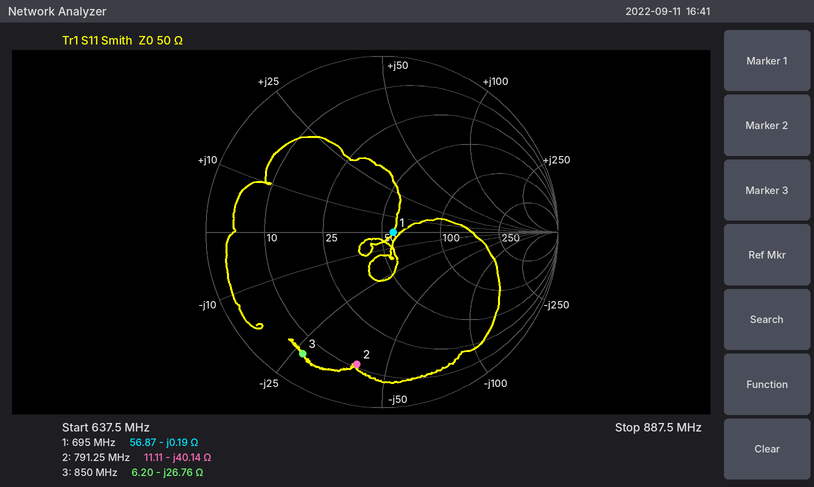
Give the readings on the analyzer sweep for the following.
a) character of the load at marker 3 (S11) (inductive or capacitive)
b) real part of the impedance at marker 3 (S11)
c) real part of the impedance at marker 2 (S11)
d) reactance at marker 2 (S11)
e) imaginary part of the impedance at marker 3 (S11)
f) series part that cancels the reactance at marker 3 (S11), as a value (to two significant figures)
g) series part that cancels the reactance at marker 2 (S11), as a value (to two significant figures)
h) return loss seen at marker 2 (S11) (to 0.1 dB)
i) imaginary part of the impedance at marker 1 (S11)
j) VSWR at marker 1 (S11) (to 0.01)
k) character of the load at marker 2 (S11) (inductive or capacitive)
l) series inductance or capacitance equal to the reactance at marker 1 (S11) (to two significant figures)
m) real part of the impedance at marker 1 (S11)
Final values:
capacitive
6.20 Ω
11.11 Ω
-40.14 Ω
-26.76 Ω
5.0 nH
8.1 nH
2.3 dB
-0.19 Ω
1.14
capacitive
1.2 nF
56.87 Ω
